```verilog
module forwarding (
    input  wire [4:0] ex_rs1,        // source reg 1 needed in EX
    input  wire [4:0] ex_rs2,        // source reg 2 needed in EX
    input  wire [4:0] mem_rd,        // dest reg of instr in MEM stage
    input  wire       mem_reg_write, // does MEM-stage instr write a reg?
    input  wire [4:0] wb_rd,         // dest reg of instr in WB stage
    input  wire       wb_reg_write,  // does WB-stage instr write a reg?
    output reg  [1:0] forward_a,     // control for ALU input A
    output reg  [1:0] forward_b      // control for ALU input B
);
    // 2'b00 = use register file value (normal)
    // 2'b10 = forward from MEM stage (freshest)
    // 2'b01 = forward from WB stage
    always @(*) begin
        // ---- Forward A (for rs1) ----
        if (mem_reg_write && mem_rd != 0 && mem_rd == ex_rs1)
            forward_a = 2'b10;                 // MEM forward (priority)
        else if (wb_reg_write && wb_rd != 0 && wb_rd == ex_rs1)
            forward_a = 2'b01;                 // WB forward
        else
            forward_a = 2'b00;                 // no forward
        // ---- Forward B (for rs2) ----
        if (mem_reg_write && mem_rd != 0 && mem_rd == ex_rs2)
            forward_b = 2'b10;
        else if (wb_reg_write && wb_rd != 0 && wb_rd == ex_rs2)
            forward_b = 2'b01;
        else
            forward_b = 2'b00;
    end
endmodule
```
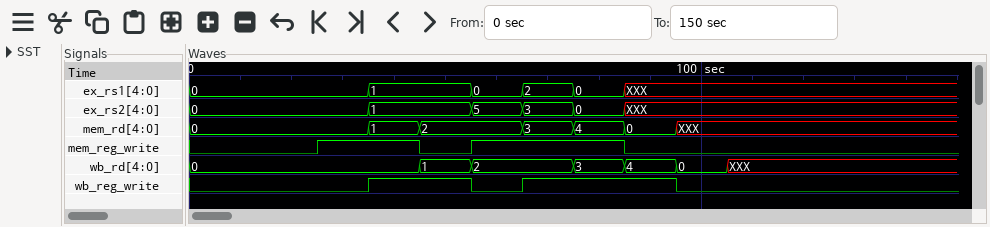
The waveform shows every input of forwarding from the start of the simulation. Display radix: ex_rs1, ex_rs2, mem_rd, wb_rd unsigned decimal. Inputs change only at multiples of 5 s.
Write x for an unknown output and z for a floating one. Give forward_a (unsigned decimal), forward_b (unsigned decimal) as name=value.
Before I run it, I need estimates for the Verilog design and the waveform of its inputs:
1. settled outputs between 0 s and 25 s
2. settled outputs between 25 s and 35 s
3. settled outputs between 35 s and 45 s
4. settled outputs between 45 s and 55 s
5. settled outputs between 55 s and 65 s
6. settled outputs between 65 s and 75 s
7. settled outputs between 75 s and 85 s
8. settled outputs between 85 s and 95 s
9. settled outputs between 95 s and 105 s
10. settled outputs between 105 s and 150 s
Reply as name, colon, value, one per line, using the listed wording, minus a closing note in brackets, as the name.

settled outputs between 0 s and 25 s: forward_a=0, forward_b=0
settled outputs between 25 s and 35 s: forward_a=0, forward_b=0
settled outputs between 35 s and 45 s: forward_a=2, forward_b=2
settled outputs between 45 s and 55 s: forward_a=1, forward_b=1
settled outputs between 55 s and 65 s: forward_a=0, forward_b=0
settled outputs between 65 s and 75 s: forward_a=1, forward_b=2
settled outputs between 75 s and 85 s: forward_a=0, forward_b=0
settled outputs between 85 s and 95 s: forward_a=0, forward_b=0
settled outputs between 95 s and 105 s: forward_a=0, forward_b=0
settled outputs between 105 s and 150 s: forward_a=0, forward_b=0
